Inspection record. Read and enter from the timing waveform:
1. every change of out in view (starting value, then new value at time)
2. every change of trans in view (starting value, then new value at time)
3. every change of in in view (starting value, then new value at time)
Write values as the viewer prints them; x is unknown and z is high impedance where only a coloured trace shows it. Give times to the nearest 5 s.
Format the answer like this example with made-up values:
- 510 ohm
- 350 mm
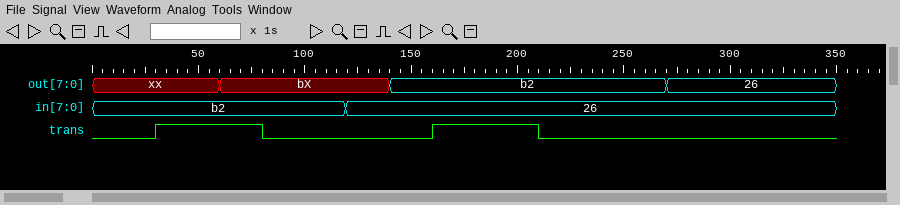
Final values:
- xx, bX at 60 s, b2 at 140 s, 26 at 270 s
- 0, 1 at 30 s, 0 at 80 s, 1 at 160 s, 0 at 210 s
- b2, 26 at 120 s
